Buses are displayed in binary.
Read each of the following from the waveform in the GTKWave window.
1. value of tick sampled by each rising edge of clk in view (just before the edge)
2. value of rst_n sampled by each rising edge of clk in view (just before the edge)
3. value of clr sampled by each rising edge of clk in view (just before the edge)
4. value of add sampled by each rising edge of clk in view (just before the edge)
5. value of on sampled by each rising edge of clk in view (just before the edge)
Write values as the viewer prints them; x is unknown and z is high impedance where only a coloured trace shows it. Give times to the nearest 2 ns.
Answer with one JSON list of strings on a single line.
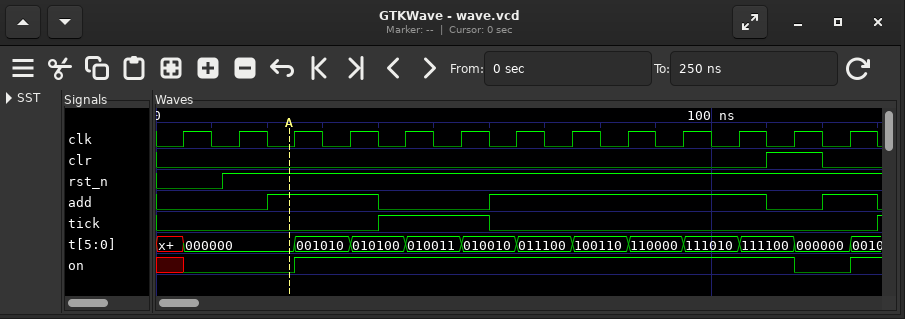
["0 0 0 0 1 1 0 0 0 0 0 0 0", "0 1 1 1 1 1 1 1 1 1 1 1 1", "0 0 0 0 0 0 0 0 0 0 0 1 0", "0 0 1 1 0 0 1 1 1 1 1 0 1", "x 0 0 1 1 1 1 1 1 1 1 1 0"]
